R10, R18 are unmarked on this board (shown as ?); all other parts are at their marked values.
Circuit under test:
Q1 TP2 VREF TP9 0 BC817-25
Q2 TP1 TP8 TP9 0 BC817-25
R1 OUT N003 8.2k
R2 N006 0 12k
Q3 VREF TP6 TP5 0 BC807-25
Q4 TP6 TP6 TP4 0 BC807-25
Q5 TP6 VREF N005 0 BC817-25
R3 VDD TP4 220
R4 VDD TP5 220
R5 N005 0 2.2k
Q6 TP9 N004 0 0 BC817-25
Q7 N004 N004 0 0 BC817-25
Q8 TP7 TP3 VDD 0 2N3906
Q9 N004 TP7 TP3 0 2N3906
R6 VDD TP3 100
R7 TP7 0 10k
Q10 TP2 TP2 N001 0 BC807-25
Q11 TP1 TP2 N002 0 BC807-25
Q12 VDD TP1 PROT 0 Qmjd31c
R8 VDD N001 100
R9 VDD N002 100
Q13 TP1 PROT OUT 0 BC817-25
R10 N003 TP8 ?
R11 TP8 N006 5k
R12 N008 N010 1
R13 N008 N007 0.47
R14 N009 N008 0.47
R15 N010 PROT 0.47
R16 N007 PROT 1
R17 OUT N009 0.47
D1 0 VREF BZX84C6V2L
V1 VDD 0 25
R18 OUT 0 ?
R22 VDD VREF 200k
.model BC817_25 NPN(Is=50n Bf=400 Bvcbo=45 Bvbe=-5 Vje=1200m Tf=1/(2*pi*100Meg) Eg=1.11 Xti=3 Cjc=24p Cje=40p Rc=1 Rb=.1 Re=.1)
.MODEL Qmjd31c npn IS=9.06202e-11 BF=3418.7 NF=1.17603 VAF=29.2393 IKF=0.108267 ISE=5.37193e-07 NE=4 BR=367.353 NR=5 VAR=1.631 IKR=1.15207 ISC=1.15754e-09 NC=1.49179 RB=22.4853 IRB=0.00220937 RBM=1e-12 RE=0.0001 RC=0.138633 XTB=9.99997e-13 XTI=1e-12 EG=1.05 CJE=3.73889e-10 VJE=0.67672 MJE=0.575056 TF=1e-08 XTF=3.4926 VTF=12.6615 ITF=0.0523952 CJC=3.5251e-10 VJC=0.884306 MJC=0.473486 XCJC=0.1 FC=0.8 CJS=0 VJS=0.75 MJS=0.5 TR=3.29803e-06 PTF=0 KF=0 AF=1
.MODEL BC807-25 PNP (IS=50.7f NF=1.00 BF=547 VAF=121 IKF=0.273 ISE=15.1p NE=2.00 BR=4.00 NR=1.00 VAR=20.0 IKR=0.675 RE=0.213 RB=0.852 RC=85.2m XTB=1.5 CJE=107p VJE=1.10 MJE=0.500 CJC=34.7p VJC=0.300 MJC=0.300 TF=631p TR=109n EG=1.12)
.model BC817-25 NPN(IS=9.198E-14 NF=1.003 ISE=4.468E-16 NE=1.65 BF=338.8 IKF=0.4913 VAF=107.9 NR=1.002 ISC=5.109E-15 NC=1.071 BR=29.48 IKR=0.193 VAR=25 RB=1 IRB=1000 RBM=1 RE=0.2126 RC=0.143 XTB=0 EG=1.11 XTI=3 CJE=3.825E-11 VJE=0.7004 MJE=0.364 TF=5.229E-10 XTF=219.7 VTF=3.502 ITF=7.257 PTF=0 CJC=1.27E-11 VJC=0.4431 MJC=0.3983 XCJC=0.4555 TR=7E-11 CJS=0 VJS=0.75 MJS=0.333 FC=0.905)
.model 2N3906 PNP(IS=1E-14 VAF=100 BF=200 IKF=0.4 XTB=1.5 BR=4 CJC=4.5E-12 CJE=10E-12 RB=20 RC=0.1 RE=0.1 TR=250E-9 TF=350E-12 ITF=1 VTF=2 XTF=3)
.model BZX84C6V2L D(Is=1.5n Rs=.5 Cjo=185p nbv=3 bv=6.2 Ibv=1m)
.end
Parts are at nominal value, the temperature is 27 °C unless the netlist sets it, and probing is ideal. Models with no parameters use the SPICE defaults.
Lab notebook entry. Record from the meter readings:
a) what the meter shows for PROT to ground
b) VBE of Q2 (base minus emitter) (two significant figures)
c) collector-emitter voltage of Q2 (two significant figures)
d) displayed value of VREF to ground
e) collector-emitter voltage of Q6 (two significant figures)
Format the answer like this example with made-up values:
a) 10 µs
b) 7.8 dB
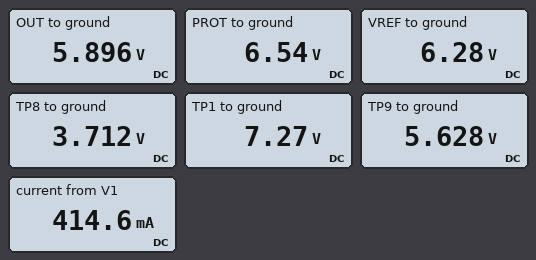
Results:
a) 6.54 V
b) -1.9 V
c) 1.6 V
d) 6.28 V
e) 5.6 V
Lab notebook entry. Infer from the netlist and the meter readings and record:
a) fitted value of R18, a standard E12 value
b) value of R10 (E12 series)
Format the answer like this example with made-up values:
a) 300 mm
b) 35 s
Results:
a) 15 Ω
b) 1.8 kΩ
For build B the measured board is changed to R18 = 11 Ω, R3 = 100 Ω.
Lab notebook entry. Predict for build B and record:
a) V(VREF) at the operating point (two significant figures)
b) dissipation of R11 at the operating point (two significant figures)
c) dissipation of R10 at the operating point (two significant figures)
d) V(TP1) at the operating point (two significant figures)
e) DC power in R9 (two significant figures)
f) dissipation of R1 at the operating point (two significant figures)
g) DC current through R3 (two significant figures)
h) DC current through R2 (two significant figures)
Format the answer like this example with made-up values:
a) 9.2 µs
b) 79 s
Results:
a) 6.2 V
b) 130 µW
c) 46 µW
d) 5.7 V
e) 4.9 mW
f) 210 µW
g) 2.5 mA
h) 160 µA
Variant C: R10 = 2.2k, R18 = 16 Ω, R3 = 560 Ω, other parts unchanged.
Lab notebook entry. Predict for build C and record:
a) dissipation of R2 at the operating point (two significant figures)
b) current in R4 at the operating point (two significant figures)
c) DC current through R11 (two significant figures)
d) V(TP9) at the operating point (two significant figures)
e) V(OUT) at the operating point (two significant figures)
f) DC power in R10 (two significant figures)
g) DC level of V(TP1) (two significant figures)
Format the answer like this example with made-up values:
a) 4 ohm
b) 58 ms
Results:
a) 630 µW
b) 6.5 mA
c) 230 µA
d) 5.7 V
e) 6.3 V
f) 120 µW
g) 7.7 V
